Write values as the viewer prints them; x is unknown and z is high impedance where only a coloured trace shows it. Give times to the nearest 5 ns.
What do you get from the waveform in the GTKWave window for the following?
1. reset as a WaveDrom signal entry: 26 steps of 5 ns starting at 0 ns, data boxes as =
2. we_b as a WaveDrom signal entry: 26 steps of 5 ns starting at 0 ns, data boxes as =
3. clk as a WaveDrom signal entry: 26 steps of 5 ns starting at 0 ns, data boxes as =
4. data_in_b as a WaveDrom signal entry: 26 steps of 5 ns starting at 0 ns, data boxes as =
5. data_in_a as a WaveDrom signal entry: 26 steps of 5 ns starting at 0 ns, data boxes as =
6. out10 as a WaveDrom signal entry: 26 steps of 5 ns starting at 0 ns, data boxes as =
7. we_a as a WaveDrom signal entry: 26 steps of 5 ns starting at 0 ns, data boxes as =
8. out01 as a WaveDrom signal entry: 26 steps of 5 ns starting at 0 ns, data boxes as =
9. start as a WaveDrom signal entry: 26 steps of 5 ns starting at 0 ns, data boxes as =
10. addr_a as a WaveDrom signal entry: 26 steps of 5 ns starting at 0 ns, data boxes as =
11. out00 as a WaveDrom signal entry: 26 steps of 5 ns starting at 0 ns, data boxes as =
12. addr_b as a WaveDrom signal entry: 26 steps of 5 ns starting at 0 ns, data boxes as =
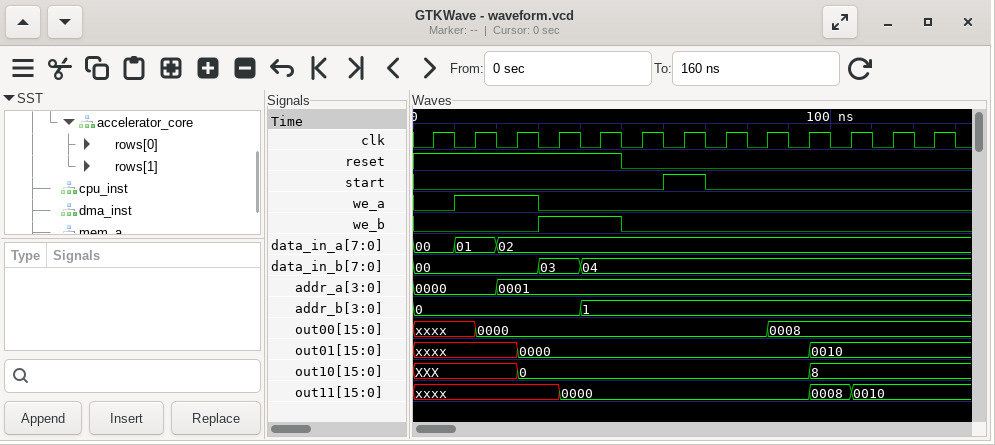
{name: 'reset', wave: '1.........0...............'}
{name: 'we_b', wave: '0.....1...0...............'}
{name: 'clk', wave: '01010101010101010101010101'}
{name: 'data_in_b', wave: '=.....=.=.................', data: '00 03 04'}
{name: 'data_in_a', wave: '=.=.=.....................', data: '00 01 02'}
{name: 'out10', wave: 'x....=.............=......', data: '0 8'}
{name: 'we_a', wave: '0.1...0...................'}
{name: 'out01', wave: 'x....=.............=......', data: '0000 0010'}
{name: 'start', wave: '0...........1.0...........'}
{name: 'addr_a', wave: '=...=.....................', data: '0000 0001'}
{name: 'out00', wave: 'x..=.............=........', data: '0000 0008'}
{name: 'addr_b', wave: '=.......=.................', data: '0 1'}
